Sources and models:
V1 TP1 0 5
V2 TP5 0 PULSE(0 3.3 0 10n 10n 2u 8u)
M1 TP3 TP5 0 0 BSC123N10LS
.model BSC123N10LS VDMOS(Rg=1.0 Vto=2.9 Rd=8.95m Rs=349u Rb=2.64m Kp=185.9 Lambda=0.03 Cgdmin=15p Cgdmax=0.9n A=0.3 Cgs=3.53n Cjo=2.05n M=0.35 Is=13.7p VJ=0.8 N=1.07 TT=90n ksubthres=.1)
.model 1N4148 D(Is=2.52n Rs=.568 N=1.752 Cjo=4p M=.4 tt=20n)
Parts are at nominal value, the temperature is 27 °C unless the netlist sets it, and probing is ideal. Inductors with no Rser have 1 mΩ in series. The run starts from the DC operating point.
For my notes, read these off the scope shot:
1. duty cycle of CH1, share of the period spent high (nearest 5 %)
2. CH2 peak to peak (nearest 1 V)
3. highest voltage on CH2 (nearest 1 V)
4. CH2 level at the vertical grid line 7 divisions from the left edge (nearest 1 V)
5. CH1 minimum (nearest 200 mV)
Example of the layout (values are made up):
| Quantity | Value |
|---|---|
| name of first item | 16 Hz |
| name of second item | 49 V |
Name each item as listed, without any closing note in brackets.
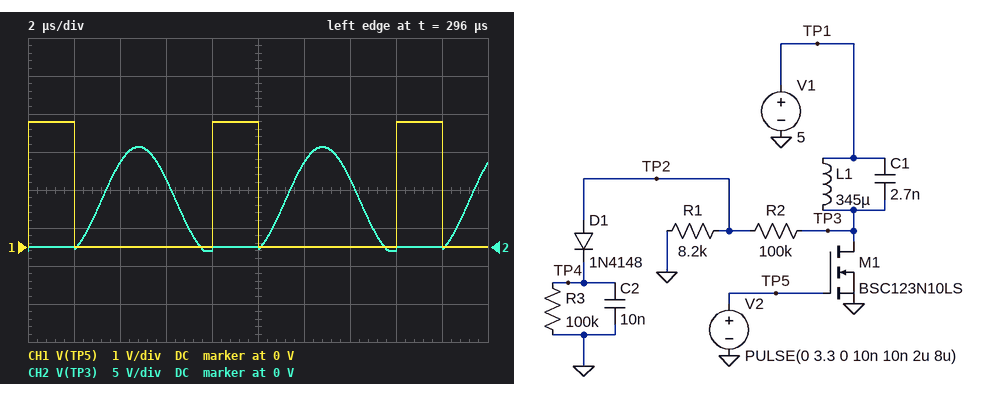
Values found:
| Quantity | Value |
|---|---|
| duty cycle of CH1, share of the period spent high | 25 % |
| CH2 peak to peak | 14 V |
| highest voltage on CH2 | 13 V |
| CH2 level at the vertical grid line 7 divisions from the left edge | 9 V |
| CH1 minimum | 0 V |
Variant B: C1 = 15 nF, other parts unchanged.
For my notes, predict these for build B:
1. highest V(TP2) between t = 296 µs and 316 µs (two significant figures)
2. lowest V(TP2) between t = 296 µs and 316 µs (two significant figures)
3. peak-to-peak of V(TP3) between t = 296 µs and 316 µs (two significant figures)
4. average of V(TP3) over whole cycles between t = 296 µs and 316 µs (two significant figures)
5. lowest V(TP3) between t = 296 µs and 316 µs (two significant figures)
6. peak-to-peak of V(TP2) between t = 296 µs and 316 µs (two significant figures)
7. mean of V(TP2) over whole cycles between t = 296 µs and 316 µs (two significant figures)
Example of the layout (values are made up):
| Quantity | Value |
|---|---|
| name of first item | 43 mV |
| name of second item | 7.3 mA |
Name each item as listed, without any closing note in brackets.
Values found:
| Quantity | Value |
|---|---|
| highest V(TP2) between t = 296 µs and 316 µs | 690 mV |
| lowest V(TP2) between t = 296 µs and 316 µs | -3.9 mV |
| peak-to-peak of V(TP3) between t = 296 µs and 316 µs | 12 V |
| average of V(TP3) over whole cycles between t = 296 µs and 316 µs | 5.0 V |
| lowest V(TP3) between t = 296 µs and 316 µs | -87 mV |
| peak-to-peak of V(TP2) between t = 296 µs and 316 µs | 700 mV |
| mean of V(TP2) over whole cycles between t = 296 µs and 316 µs | 340 mV |
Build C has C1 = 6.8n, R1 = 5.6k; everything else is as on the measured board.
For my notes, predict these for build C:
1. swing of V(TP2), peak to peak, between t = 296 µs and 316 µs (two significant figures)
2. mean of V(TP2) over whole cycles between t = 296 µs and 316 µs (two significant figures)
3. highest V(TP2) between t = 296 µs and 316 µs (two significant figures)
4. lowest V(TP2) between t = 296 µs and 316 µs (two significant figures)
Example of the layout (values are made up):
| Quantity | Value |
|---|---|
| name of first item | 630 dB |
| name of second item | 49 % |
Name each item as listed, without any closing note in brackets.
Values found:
| Quantity | Value |
|---|---|
| swing of V(TP2), peak to peak, between t = 296 µs and 316 µs | 530 mV |
| mean of V(TP2) over whole cycles between t = 296 µs and 316 µs | 250 mV |
| highest V(TP2) between t = 296 µs and 316 µs | 520 mV |
| lowest V(TP2) between t = 296 µs and 316 µs | -8.4 mV |
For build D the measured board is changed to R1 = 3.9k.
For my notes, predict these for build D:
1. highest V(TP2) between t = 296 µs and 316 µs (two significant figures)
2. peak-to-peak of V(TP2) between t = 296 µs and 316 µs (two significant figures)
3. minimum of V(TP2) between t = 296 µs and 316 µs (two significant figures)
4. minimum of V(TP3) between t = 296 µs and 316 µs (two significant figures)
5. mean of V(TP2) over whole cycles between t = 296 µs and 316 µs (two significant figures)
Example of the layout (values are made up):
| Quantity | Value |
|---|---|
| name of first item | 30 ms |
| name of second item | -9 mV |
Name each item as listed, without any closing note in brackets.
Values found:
| Quantity | Value |
|---|---|
| highest V(TP2) between t = 296 µs and 316 µs | 450 mV |
| peak-to-peak of V(TP2) between t = 296 µs and 316 µs | 480 mV |
| minimum of V(TP2) between t = 296 µs and 316 µs | -21 mV |
| minimum of V(TP3) between t = 296 µs and 316 µs | -570 mV |
| mean of V(TP2) over whole cycles between t = 296 µs and 316 µs | 180 mV |
